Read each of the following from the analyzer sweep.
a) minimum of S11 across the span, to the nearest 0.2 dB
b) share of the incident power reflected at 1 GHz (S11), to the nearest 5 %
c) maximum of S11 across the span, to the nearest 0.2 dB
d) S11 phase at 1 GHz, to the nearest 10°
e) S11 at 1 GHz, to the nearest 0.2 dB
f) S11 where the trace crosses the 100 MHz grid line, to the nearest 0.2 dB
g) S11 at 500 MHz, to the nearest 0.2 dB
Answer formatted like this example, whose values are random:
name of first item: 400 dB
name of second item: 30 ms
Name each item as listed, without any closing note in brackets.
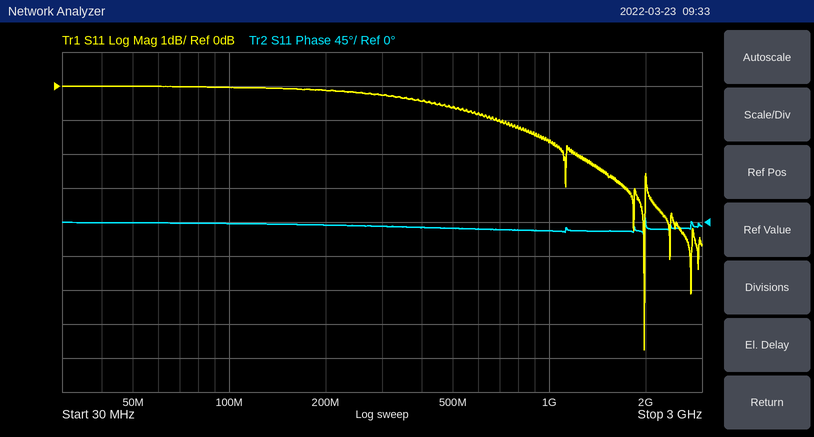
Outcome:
minimum of S11 across the span, to the nearest 0.2 dB: -7.8 dB
share of the incident power reflected at 1 GHz (S11), to the nearest 5 %: 70 %
maximum of S11 across the span, to the nearest 0.2 dB: 0.0 dB
S11 phase at 1 GHz, to the nearest 10°: -10°
S11 at 1 GHz, to the nearest 0.2 dB: -1.6 dB
S11 where the trace crosses the 100 MHz grid line, to the nearest 0.2 dB: 0.0 dB
S11 at 500 MHz, to the nearest 0.2 dB: -0.6 dB
